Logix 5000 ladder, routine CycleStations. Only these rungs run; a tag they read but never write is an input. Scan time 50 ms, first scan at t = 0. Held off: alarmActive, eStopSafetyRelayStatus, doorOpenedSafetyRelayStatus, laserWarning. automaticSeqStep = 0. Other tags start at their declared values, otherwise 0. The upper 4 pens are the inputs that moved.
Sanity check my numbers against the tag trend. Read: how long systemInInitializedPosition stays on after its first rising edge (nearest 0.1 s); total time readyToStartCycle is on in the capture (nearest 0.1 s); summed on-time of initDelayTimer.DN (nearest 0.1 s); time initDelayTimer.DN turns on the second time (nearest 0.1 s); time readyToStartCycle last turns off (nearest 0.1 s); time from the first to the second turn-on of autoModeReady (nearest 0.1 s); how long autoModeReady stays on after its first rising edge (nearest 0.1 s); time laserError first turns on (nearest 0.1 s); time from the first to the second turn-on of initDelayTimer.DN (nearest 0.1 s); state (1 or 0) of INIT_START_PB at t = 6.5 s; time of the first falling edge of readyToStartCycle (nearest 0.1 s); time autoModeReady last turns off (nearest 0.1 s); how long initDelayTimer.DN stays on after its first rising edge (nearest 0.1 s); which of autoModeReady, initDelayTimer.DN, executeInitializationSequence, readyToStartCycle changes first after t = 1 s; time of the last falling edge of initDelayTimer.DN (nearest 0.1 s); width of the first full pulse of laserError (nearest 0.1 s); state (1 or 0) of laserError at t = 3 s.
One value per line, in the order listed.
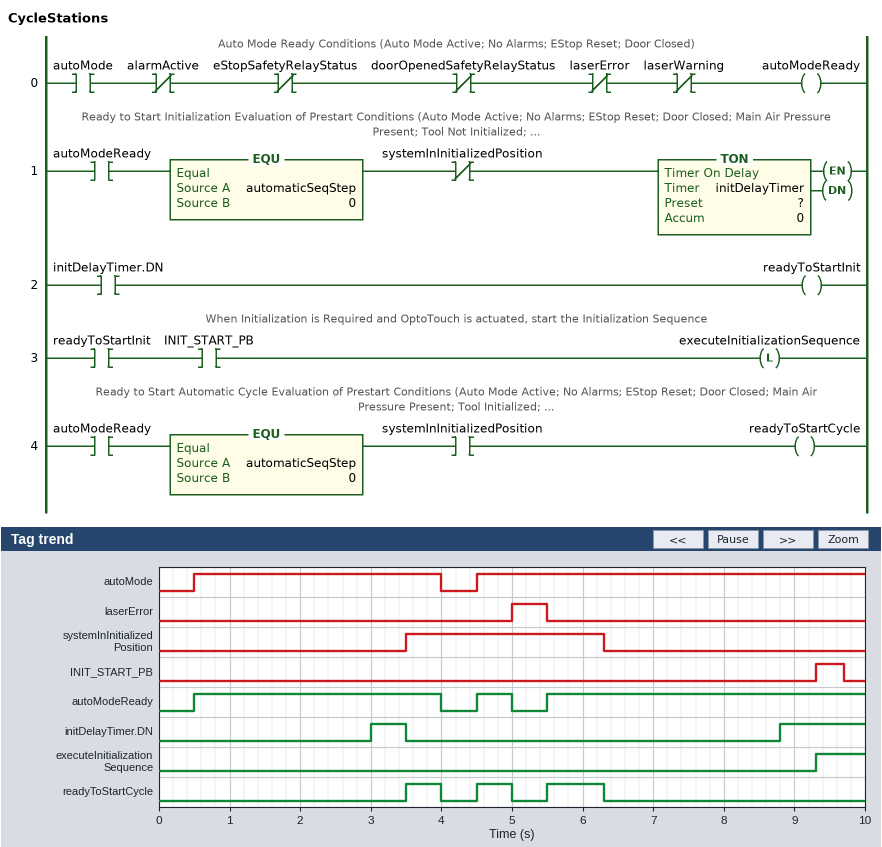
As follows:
2.8 s
1.8 s
1.7 s
8.8 s
6.3 s
4.0 s
3.5 s
5.0 s
5.8 s
0
4.0 s
5.0 s
0.5 s
initDelayTimer.DN
3.5 s
0.5 s
0
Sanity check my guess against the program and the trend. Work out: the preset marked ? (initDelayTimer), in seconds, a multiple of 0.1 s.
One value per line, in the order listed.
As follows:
2.5 s
